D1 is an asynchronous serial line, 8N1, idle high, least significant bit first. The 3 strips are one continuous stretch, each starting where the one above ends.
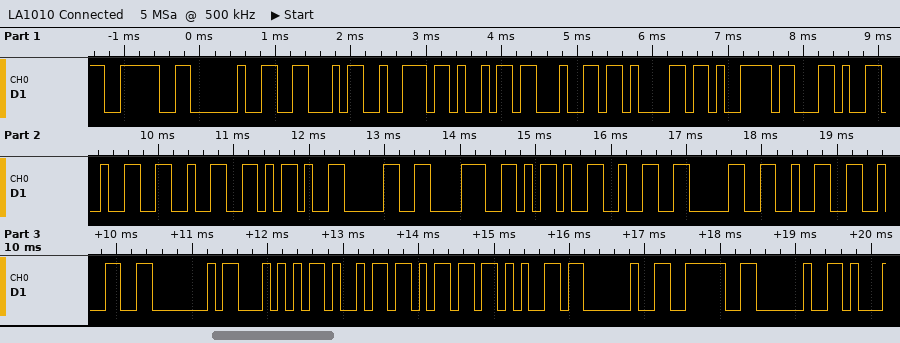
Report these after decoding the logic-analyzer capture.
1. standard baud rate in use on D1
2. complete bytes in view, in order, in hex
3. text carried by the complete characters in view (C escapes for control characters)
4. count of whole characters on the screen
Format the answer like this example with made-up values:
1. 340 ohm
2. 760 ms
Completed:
1. 9600 baud
2. 3E 20 46 72 69 64 61 79 2C 32 32 2D 30 38 2D 32 30 32 32 40 54 69 6D 65 20 3E 20
3. "> Friday,22-08-2022@Time > "
4. 27
